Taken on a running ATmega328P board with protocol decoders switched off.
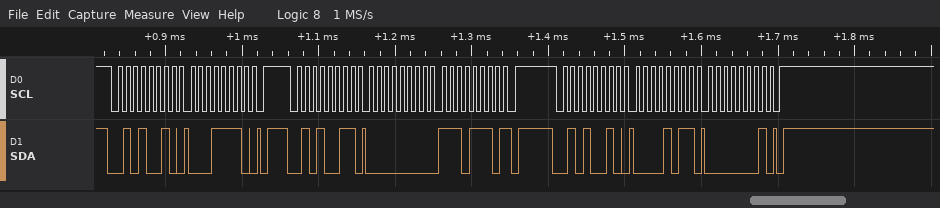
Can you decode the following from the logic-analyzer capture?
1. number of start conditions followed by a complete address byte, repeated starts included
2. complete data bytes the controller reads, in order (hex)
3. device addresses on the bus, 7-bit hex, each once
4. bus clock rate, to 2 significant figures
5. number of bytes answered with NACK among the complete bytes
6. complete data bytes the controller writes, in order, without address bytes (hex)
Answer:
3
00 EE
0x29
100 kHz
1
1E 0B 01
